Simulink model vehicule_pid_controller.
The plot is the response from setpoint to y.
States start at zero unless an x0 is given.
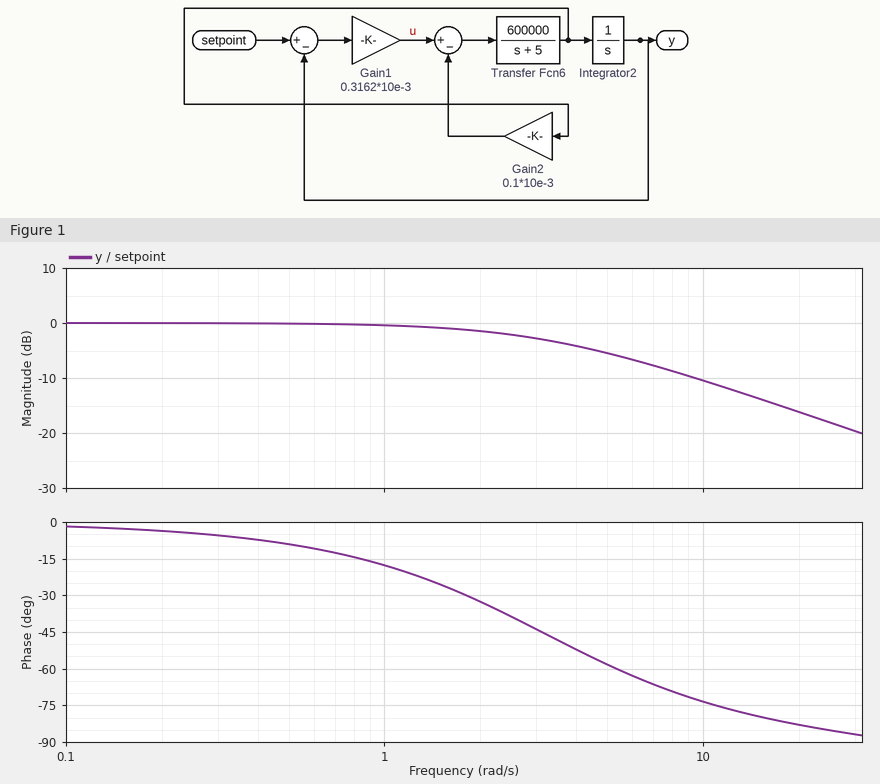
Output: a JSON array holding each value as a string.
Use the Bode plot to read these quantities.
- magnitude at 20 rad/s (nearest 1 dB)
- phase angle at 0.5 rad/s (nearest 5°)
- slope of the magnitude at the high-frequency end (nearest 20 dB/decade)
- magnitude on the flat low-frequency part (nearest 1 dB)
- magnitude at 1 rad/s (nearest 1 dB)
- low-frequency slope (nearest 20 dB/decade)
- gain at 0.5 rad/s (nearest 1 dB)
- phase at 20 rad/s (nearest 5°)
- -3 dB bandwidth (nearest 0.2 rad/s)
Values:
["-16 dB", "-10°", "-20 dB/decade", "0 dB", "0 dB", "0 dB/decade", "0 dB", "-85°", "3.2 rad/s"]
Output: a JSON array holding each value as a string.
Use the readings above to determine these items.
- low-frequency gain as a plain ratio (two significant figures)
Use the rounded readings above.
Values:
["1.0"]
